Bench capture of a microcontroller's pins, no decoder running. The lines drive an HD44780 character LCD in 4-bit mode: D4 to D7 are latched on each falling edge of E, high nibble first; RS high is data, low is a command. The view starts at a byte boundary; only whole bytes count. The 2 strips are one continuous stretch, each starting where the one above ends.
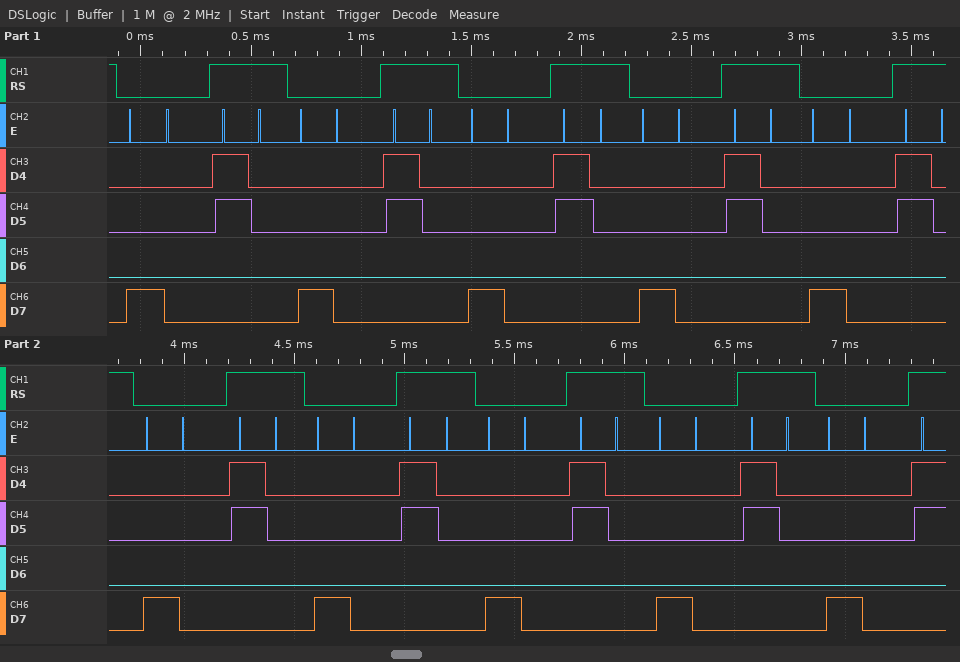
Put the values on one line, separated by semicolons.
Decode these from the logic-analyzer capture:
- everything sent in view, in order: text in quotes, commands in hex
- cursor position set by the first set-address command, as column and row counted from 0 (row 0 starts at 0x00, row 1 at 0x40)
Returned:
0x80 "0" 0x80 "0" 0x80 "0" 0x80 "0" 0x80 "0" 0x80 "0" 0x80 "0" 0x80 "0" 0x80 "0" 0x80; column 0, row 0
